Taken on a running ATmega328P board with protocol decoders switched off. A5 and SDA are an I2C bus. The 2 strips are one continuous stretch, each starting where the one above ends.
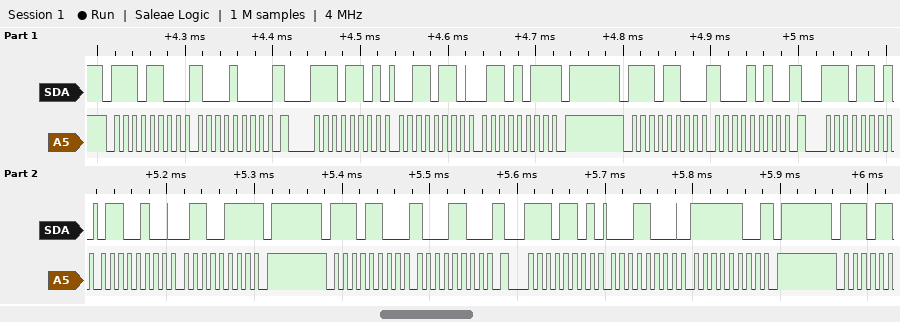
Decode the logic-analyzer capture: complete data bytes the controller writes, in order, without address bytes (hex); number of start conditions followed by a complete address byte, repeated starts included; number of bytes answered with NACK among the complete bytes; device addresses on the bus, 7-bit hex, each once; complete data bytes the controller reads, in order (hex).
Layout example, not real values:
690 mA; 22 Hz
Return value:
88 8A 8C; 6; 3; 0x76; 36 6B 64 67 18 FC
